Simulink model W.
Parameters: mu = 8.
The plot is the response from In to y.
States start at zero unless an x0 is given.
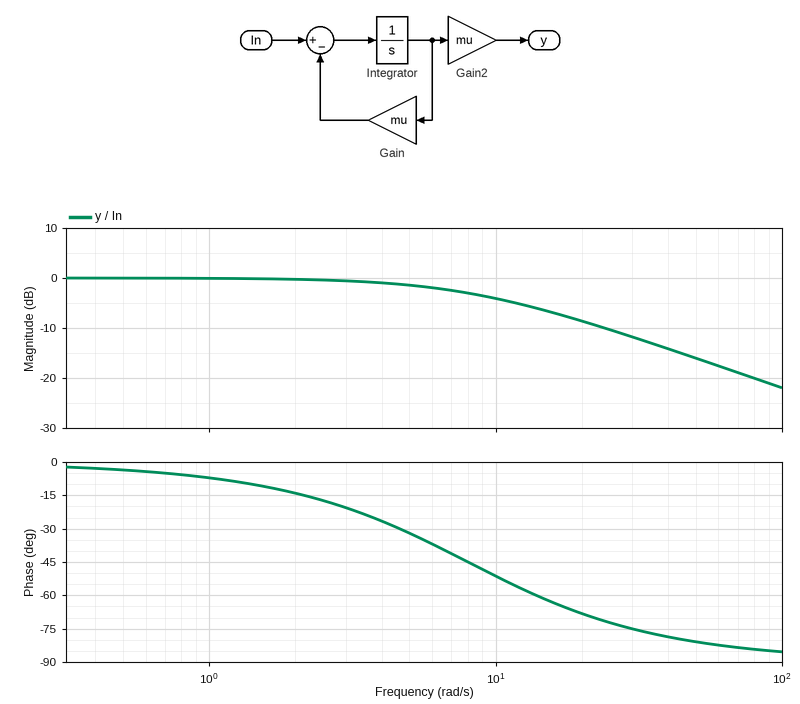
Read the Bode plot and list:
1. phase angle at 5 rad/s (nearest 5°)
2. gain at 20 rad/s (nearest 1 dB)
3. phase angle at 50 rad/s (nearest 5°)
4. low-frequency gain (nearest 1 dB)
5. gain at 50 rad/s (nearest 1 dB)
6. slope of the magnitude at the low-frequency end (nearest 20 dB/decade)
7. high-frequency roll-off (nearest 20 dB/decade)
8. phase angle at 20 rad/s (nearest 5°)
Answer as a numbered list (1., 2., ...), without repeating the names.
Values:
1. -30°
2. -9 dB
3. -80°
4. 0 dB
5. -16 dB
6. 0 dB/decade
7. -20 dB/decade
8. -70°
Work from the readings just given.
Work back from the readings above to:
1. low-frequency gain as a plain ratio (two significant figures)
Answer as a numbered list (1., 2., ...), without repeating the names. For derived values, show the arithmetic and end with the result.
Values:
1. 10^(0 / 20) = 1.0
